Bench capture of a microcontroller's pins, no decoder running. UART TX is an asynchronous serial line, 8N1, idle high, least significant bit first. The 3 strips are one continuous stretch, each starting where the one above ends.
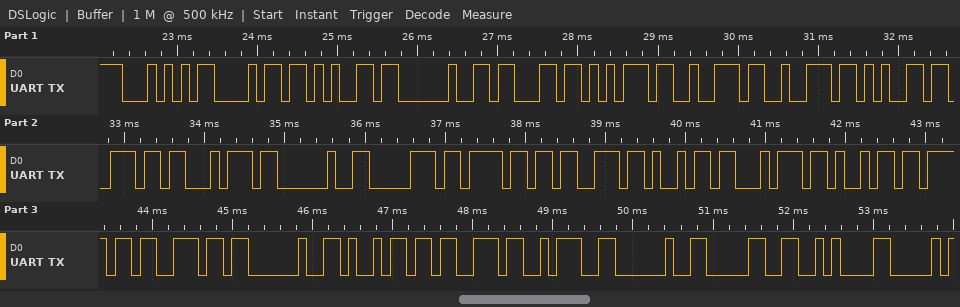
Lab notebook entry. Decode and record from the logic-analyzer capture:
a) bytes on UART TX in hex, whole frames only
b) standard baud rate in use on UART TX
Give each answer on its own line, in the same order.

54 68 65 20 63 75 72 72 65 6E 74 20 70 6F 73 69 74 69 6F 6E 20 69 73 3A 20 30 0A
9600 baud
